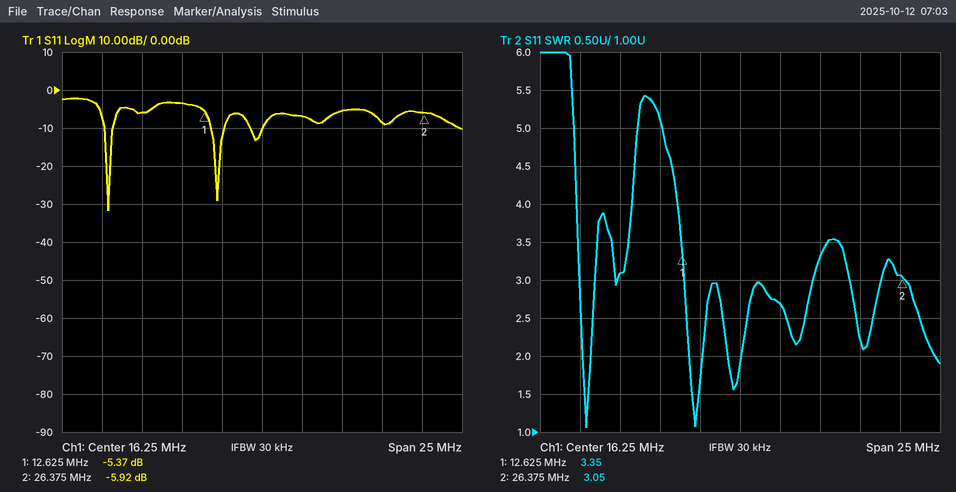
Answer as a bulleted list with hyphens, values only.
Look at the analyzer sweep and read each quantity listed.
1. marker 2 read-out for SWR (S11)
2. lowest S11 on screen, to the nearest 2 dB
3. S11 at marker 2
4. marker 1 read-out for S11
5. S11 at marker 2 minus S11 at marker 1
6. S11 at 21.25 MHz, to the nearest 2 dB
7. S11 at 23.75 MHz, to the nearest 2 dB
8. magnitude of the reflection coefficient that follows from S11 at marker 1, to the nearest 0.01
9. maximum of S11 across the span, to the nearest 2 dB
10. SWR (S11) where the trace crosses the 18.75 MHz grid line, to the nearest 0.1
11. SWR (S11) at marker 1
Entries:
- 3.05
- -32 dB
- -5.92 dB
- -5.37 dB
- -0.55 dB
- -6 dB
- -8 dB
- 0.54
- -2 dB
- 2.7
- 3.35
